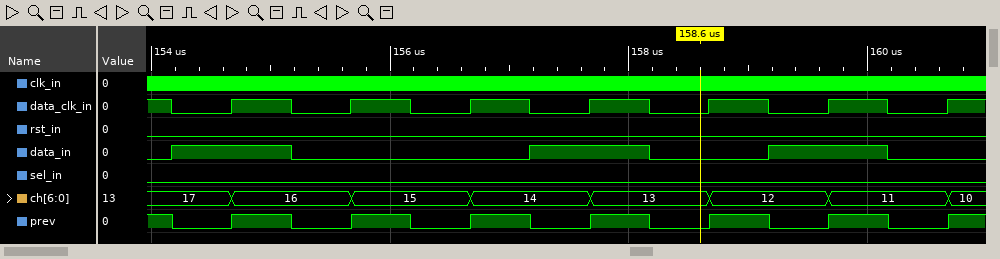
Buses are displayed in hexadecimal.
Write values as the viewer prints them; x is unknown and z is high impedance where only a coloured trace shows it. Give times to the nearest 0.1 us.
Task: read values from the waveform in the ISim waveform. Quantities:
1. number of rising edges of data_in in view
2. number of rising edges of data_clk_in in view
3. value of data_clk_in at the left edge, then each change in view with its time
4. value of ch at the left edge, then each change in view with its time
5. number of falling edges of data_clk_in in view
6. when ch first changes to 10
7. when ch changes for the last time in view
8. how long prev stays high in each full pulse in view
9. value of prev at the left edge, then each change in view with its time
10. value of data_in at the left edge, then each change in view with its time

3
7
1, 0 at 154.2 us, 1 at 154.7 us, 0 at 155.2 us, 1 at 155.7 us, 0 at 156.2 us, 1 at 156.7 us, 0 at 157.2 us, 1 at 157.7 us, 0 at 158.2 us, 1 at 158.7 us, 0 at 159.2 us, 1 at 159.7 us, 0 at 160.2 us, 1 at 160.7 us
17, 16 at 154.7 us, 15 at 155.7 us, 14 at 156.7 us, 13 at 157.7 us, 12 at 158.7 us, 11 at 159.7 us, 10 at 160.7 us
7
160.7 us
160.7 us
0.5 us, 0.5 us, 0.5 us, 0.5 us, 0.5 us, 0.5 us
1, 0 at 154.2 us, 1 at 154.7 us, 0 at 155.2 us, 1 at 155.7 us, 0 at 156.2 us, 1 at 156.7 us, 0 at 157.2 us, 1 at 157.7 us, 0 at 158.2 us, 1 at 158.7 us, 0 at 159.2 us, 1 at 159.7 us, 0 at 160.2 us, 1 at 160.7 us
0, 1 at 154.2 us, 0 at 155.2 us, 1 at 157.2 us, 0 at 158.2 us, 1 at 159.2 us, 0 at 160.2 us
